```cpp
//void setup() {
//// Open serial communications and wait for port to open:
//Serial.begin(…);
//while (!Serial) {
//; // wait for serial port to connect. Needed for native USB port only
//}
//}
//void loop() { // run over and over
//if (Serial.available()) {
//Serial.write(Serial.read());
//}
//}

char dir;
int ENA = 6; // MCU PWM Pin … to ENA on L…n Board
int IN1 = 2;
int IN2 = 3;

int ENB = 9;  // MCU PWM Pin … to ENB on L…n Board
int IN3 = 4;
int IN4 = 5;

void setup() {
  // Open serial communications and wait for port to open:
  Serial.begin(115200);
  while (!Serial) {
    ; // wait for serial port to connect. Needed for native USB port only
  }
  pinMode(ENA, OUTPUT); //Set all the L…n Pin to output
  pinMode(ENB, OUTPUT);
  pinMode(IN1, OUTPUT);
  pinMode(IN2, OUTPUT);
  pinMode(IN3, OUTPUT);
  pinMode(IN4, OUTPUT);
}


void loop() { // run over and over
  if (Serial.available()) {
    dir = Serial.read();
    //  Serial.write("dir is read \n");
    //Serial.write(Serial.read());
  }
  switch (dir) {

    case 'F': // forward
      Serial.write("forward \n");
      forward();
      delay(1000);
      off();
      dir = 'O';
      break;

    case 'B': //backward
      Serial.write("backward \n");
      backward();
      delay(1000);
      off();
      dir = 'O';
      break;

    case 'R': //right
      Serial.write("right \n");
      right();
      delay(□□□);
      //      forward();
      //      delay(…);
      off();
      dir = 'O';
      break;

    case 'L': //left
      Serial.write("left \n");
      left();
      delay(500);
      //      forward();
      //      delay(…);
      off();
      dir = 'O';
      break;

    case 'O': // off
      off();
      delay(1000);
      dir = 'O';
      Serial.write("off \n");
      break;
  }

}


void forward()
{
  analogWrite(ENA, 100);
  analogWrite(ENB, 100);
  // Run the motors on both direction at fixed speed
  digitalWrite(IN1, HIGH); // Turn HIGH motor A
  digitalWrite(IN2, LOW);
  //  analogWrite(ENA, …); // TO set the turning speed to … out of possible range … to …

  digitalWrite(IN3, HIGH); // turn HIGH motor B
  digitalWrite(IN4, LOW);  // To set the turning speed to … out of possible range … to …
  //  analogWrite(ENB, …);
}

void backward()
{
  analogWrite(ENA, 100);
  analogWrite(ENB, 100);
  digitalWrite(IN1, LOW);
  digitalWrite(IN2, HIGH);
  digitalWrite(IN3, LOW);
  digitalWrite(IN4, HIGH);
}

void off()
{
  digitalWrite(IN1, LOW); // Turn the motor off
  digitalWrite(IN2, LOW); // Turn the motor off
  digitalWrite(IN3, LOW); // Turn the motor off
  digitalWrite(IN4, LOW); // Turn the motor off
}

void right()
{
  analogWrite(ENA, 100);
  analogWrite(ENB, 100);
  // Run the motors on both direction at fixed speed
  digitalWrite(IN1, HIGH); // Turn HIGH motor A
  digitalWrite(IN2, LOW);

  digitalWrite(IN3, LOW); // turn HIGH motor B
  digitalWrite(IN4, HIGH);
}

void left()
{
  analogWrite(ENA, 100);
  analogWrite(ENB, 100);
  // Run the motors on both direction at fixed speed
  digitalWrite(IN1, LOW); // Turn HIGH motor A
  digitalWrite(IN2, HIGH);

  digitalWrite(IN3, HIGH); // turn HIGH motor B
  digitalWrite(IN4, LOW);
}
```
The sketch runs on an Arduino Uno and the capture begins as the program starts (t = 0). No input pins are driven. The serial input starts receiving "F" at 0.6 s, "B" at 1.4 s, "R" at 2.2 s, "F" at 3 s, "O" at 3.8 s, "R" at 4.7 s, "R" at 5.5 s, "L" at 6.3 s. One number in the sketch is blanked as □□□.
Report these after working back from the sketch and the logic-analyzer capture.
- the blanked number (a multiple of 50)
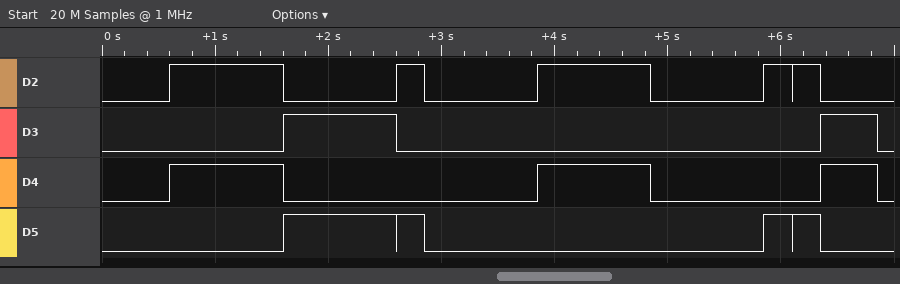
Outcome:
250
